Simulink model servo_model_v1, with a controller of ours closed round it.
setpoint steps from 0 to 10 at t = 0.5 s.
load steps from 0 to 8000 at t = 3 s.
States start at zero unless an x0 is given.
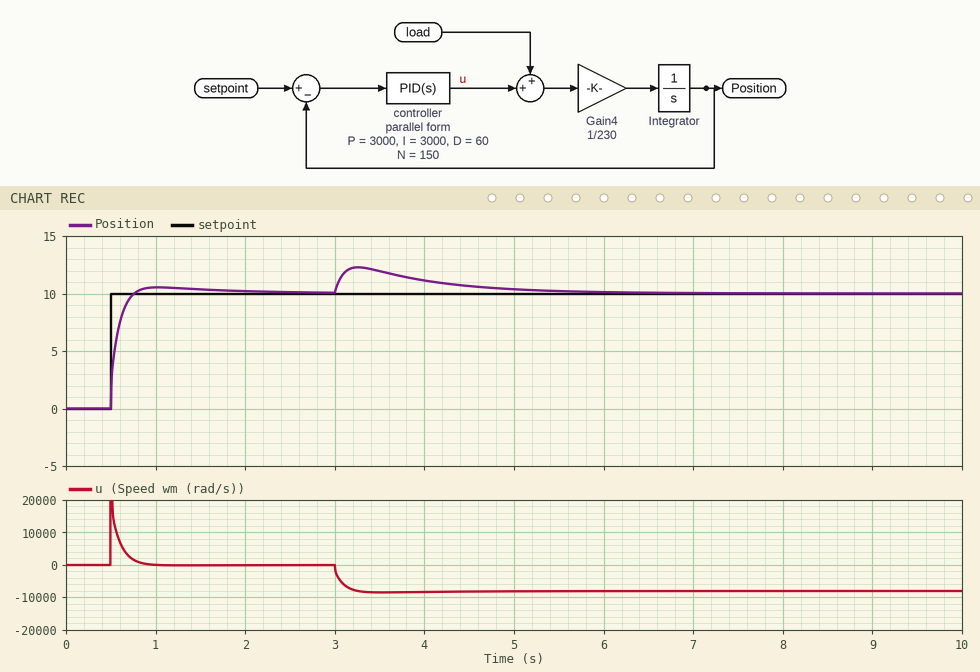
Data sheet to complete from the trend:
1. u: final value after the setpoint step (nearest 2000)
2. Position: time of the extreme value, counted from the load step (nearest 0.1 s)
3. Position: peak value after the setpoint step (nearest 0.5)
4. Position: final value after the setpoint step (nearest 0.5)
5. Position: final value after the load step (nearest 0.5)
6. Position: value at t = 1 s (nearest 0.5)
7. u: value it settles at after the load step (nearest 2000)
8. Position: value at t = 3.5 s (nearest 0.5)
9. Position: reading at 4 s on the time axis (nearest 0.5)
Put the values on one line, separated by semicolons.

0; 0.3 s; 10.5; 10.0; 10.0; 10.5; -8000; 12.0; 11.0
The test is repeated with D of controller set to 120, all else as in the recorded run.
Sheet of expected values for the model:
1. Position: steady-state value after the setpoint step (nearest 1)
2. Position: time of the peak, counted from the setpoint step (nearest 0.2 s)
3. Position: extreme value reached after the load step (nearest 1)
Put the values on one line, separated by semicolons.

10; 0.6 s; 12
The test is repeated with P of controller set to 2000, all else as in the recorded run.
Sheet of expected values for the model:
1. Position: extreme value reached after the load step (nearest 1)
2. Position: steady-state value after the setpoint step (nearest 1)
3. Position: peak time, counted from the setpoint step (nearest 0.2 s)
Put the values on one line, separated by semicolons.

13; 10; 0.6 s
